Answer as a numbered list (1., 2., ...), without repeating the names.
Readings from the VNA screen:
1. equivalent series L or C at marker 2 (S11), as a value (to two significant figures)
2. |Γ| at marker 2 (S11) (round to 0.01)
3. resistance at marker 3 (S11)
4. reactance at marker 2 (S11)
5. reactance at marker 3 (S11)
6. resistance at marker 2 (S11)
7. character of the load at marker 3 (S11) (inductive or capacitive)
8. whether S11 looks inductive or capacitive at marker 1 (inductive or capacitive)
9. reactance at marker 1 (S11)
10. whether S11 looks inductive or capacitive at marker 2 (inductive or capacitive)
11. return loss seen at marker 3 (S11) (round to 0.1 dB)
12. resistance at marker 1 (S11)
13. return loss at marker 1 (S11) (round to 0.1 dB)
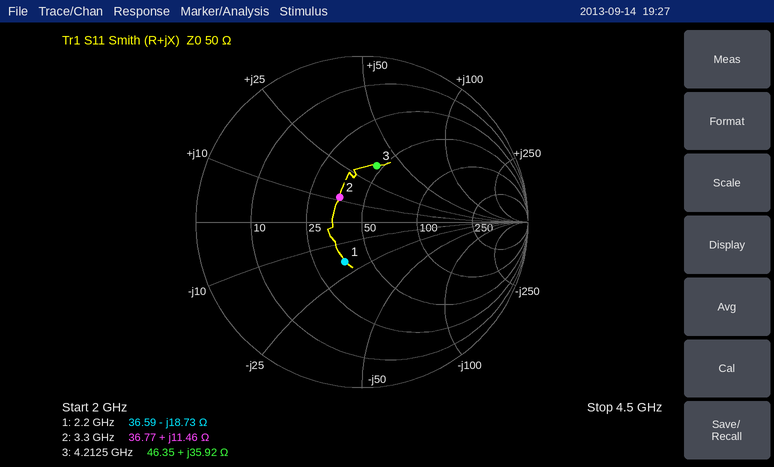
1. 550 pH
2. 0.20
3. 46.35 Ω
4. +11.46 Ω
5. +35.92 Ω
6. 36.77 Ω
7. inductive
8. capacitive
9. -18.73 Ω
10. inductive
11. 9.1 dB
12. 36.59 Ω
13. 11.7 dB
